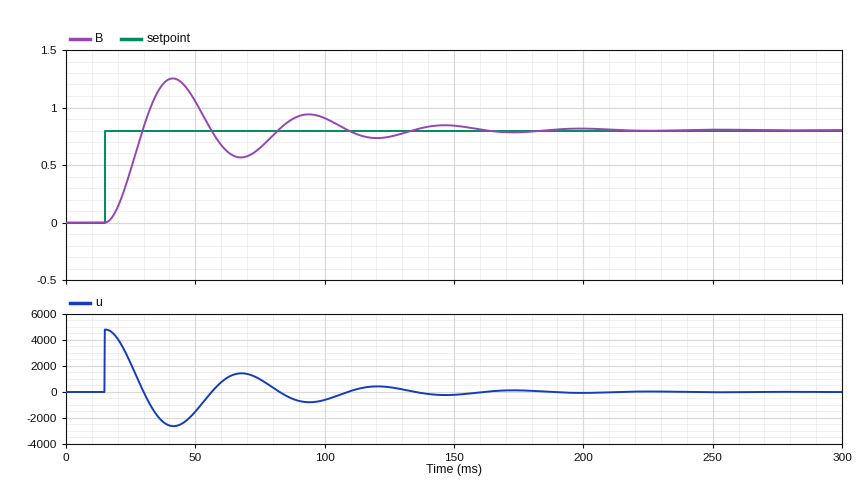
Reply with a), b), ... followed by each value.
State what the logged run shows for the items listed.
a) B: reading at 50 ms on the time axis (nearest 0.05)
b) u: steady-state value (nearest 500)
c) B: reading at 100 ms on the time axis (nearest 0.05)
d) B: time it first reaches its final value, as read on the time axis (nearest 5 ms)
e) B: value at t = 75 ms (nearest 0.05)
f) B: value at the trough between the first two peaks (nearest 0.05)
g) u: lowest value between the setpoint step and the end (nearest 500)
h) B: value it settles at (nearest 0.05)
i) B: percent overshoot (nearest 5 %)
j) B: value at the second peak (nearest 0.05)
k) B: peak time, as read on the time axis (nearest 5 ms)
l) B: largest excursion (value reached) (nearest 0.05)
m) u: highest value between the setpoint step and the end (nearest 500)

a) 1.05
b) 0
c) 0.90
d) 30 ms
e) 0.65
f) 0.55
g) -2500
h) 0.80
i) 55 %
j) 0.95
k) 40 ms
l) 1.25
m) 5000
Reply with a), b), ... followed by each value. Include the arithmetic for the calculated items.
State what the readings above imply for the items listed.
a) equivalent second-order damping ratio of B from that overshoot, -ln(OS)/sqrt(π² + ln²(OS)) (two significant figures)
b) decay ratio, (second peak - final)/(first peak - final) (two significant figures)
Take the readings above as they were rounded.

a) ln(0.55) = -0.598; 0.598 / sqrt(9.870 + 0.357) = 0.19
b) (0.95 - 0.8) / (1.25 - 0.8) = 0.33
